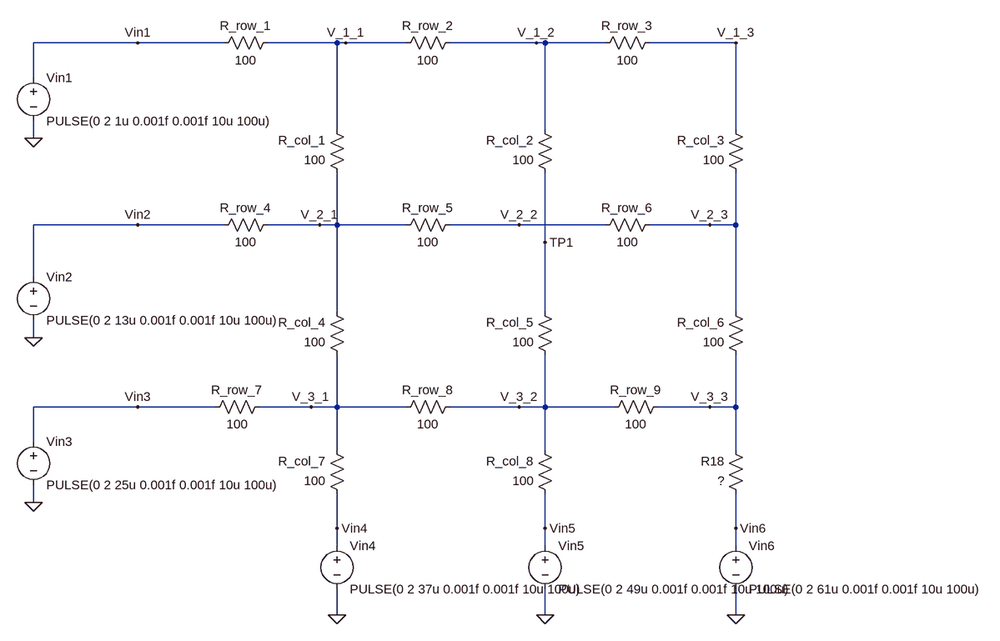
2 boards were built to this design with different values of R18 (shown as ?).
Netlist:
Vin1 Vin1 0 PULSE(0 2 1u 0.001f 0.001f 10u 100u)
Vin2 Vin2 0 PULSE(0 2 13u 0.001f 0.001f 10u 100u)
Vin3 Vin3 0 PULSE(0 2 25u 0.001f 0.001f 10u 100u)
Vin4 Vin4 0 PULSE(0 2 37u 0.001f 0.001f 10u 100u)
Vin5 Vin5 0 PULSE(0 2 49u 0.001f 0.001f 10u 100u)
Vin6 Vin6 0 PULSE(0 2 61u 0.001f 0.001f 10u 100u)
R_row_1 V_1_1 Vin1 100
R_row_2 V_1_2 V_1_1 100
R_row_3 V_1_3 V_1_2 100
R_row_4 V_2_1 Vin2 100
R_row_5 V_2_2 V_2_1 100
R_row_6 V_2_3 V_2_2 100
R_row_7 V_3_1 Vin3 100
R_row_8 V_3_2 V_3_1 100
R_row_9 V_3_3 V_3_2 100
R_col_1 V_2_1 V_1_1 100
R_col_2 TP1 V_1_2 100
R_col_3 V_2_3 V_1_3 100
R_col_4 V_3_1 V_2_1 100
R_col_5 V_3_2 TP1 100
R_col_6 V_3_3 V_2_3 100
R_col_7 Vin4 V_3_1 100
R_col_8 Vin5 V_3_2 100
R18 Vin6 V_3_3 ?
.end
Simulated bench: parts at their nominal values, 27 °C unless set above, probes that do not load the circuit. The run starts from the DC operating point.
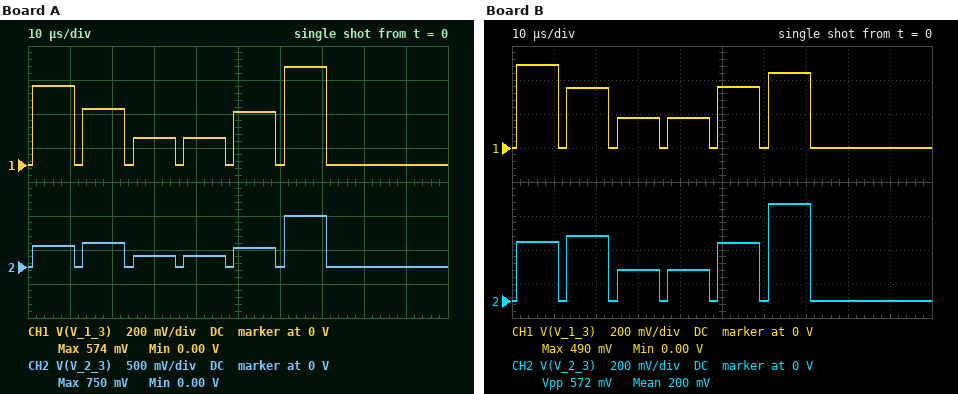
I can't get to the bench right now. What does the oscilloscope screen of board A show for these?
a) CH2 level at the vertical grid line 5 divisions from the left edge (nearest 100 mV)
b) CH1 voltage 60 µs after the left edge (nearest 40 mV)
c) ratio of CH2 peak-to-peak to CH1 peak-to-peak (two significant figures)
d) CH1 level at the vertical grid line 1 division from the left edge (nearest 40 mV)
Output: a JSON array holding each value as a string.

["300 mV", "0 V", "1.3", "480 mV"]
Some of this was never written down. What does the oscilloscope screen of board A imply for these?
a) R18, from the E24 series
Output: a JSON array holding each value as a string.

["68 Ω"]
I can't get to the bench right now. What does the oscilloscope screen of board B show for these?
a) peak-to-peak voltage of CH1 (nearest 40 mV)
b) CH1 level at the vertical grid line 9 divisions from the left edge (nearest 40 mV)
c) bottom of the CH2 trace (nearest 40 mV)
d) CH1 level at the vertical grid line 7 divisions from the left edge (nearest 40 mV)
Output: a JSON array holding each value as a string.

["480 mV", "0 V", "0 V", "440 mV"]
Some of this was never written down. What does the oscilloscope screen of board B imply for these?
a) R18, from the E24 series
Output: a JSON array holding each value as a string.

["120 Ω"]
